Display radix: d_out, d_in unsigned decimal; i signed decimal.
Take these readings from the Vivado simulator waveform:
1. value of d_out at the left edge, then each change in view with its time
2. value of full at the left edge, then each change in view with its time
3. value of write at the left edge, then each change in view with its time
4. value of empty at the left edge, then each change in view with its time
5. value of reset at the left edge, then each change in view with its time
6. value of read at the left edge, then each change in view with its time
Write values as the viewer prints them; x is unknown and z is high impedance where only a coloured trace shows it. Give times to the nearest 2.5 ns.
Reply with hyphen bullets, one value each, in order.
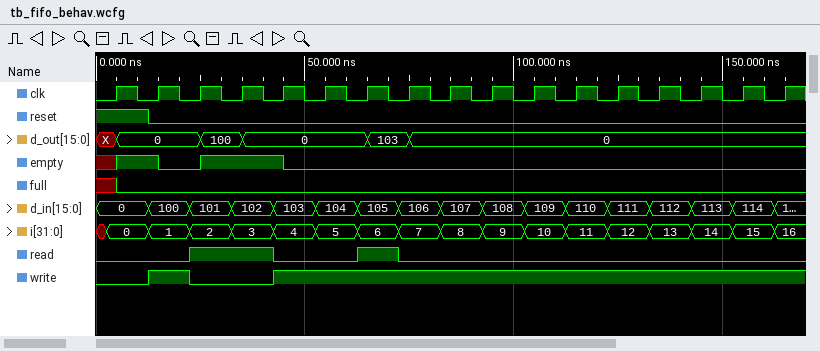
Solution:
- X, 0 at 5 ns, 100 at 25 ns, 0 at 35 ns, 103 at 65 ns, 0 at 75 ns
- x, 0 at 5 ns
- 0, 1 at 12.5 ns, 0 at 22.5 ns, 1 at 42.5 ns
- x, 1 at 5 ns, 0 at 15 ns, 1 at 25 ns, 0 at 45 ns
- 1, 0 at 12.5 ns
- 0, 1 at 22.5 ns, 0 at 42.5 ns, 1 at 62.5 ns, 0 at 72.5 ns
